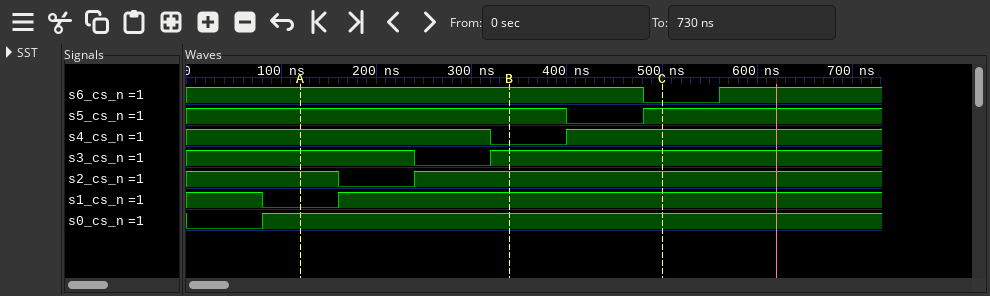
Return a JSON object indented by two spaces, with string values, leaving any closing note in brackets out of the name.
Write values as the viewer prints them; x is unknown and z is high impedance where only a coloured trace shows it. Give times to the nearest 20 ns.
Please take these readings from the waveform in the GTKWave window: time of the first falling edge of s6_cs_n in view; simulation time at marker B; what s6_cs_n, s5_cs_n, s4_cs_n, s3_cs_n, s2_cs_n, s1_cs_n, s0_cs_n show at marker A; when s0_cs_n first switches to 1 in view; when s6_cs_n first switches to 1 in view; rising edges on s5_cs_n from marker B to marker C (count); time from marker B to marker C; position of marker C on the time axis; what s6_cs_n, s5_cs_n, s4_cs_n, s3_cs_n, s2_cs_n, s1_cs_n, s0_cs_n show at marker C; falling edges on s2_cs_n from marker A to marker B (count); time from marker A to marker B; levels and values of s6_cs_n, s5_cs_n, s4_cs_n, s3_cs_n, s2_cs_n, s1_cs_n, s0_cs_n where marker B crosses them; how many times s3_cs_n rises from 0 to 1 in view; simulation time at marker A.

{
  "time of the first falling edge of s6_cs_n in view": "480 ns",
  "simulation time at marker B": "340 ns",
  "what s6_cs_n, s5_cs_n, s4_cs_n, s3_cs_n, s2_cs_n, s1_cs_n, s0_cs_n show at marker A": "s6_cs_n=1, s5_cs_n=1, s4_cs_n=1, s3_cs_n=1, s2_cs_n=1, s1_cs_n=0, s0_cs_n=1",
  "when s0_cs_n first switches to 1 in view": "80 ns",
  "when s6_cs_n first switches to 1 in view": "560 ns",
  "rising edges on s5_cs_n from marker B to marker C": "1",
  "time from marker B to marker C": "160 ns",
  "position of marker C on the time axis": "500 ns",
  "what s6_cs_n, s5_cs_n, s4_cs_n, s3_cs_n, s2_cs_n, s1_cs_n, s0_cs_n show at marker C": "s6_cs_n=0, s5_cs_n=1, s4_cs_n=1, s3_cs_n=1, s2_cs_n=1, s1_cs_n=1, s0_cs_n=1",
  "falling edges on s2_cs_n from marker A to marker B": "1",
  "time from marker A to marker B": "220 ns",
  "levels and values of s6_cs_n, s5_cs_n, s4_cs_n, s3_cs_n, s2_cs_n, s1_cs_n, s0_cs_n where marker B crosses them": "s6_cs_n=1, s5_cs_n=1, s4_cs_n=0, s3_cs_n=1, s2_cs_n=1, s1_cs_n=1, s0_cs_n=1",
  "how many times s3_cs_n rises from 0 to 1 in view": "1",
  "simulation time at marker A": "120 ns"
}
